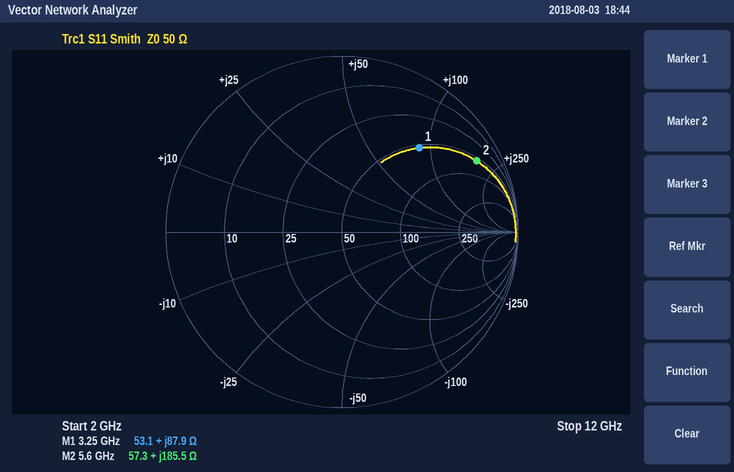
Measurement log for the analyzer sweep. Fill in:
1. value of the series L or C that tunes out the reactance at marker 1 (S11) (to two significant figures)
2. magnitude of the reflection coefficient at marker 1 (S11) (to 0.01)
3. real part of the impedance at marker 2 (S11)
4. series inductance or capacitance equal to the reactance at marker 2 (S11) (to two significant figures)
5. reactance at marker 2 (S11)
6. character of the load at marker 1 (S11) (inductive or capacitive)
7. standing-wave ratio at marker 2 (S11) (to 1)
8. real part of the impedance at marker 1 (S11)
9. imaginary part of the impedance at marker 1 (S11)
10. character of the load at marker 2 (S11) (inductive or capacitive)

560 fF
0.65
57.3 Ω
5.3 nH
+185.5 Ω
inductive
14
53.1 Ω
+87.9 Ω
inductive
